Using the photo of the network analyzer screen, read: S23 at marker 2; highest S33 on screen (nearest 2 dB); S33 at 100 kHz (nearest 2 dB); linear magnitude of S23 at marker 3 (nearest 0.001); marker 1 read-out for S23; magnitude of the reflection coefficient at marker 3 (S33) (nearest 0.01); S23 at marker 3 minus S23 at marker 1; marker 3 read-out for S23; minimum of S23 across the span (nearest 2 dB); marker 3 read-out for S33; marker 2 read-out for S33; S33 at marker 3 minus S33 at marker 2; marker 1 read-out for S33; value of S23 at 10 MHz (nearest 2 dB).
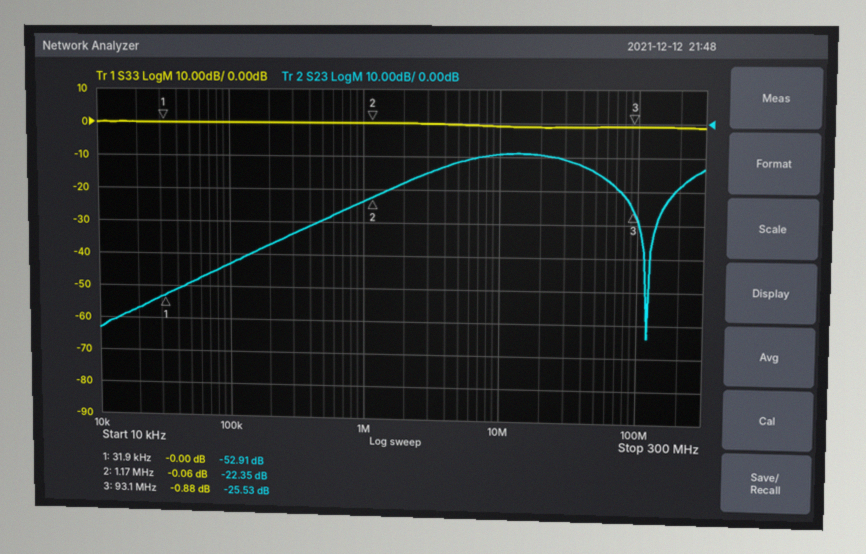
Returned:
-22.35 dB
0 dB
0 dB
0.053
-52.91 dB
0.90
27.38 dB
-25.53 dB
-64 dB
-0.88 dB
-0.06 dB
-0.82 dB
-0.00 dB
-10 dB
